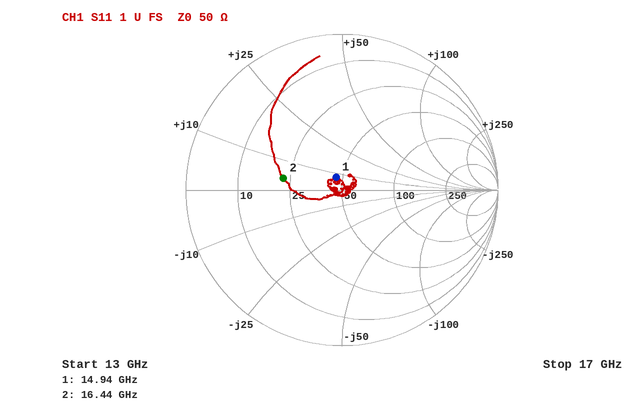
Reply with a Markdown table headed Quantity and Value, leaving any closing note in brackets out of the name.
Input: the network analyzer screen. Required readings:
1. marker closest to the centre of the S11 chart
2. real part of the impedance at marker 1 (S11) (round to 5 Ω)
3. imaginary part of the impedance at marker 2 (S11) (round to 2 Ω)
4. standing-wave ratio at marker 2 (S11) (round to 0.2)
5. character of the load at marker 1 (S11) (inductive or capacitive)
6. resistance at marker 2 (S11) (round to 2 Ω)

| Quantity | Value |
|---|---|
| marker closest to the centre of the S11 chart | marker 1 |
| real part of the impedance at marker 1 (S11) | 45 Ω |
| imaginary part of the impedance at marker 2 (S11) | +4 Ω |
| standing-wave ratio at marker 2 (S11) | 2.2 |
| character of the load at marker 1 (S11) | inductive |
| resistance at marker 2 (S11) | 22 Ω |
